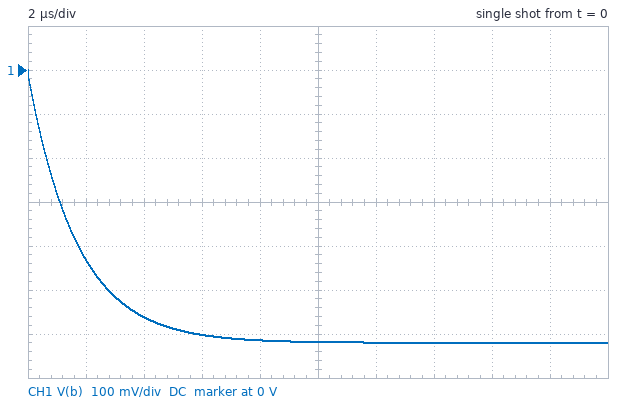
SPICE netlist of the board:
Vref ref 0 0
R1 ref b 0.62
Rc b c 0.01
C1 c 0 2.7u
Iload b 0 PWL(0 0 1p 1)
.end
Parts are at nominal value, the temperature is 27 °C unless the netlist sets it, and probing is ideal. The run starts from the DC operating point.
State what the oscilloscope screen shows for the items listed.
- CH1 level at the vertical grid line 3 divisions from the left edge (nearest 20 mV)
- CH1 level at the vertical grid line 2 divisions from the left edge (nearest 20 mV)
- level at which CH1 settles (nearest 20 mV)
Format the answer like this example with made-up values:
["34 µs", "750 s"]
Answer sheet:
["-600 mV", "-560 mV", "-620 mV"]
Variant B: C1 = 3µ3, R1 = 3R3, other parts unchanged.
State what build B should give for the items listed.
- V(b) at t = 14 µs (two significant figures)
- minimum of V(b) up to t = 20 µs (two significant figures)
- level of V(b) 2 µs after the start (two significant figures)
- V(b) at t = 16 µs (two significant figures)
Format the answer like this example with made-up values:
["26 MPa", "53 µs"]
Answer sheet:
["-2.4 V", "-2.8 V", "-560 mV", "-2.5 V"]
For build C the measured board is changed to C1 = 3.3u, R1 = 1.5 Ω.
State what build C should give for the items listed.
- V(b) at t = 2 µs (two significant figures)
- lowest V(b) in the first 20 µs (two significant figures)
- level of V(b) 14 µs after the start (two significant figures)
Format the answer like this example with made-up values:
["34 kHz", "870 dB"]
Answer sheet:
["-500 mV", "-1.5 V", "-1.4 V"]
